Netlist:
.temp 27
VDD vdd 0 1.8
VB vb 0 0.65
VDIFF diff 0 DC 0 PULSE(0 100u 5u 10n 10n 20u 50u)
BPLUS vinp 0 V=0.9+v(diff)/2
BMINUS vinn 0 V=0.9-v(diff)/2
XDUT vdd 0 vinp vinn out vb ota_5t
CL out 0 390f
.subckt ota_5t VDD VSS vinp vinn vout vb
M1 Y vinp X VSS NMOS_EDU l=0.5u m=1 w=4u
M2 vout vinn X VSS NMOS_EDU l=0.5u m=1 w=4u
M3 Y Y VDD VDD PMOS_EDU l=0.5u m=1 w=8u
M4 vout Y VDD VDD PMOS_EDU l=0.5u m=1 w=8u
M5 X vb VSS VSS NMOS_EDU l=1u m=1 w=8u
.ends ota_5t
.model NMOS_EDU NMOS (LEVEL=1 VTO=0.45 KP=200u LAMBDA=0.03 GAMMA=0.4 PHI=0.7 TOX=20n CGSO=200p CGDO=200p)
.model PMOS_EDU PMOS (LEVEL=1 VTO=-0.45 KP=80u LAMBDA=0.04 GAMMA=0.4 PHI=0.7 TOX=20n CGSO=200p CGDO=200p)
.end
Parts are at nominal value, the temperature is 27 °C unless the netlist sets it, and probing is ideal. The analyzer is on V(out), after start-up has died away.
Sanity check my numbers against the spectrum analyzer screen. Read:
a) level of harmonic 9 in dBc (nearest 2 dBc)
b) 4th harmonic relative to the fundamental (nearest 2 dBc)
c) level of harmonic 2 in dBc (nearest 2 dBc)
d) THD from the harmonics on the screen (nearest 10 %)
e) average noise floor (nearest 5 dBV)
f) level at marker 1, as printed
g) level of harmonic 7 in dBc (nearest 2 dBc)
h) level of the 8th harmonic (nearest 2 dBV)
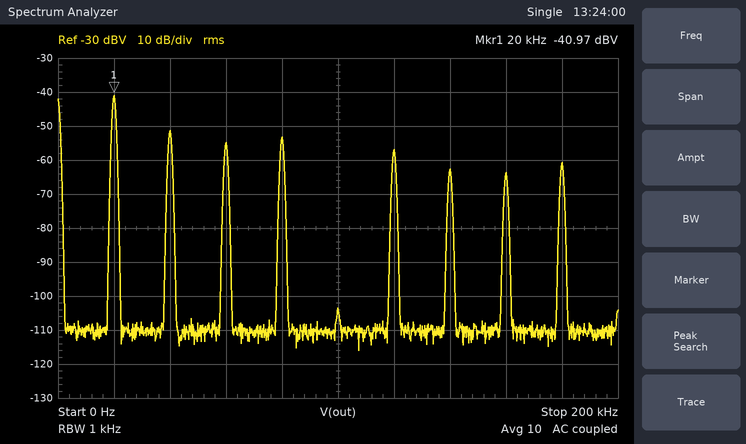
-20 dBc
-12 dBc
-10 dBc
50 %
-110 dBV
-40.97 dBV
-22 dBc
-64 dBV
